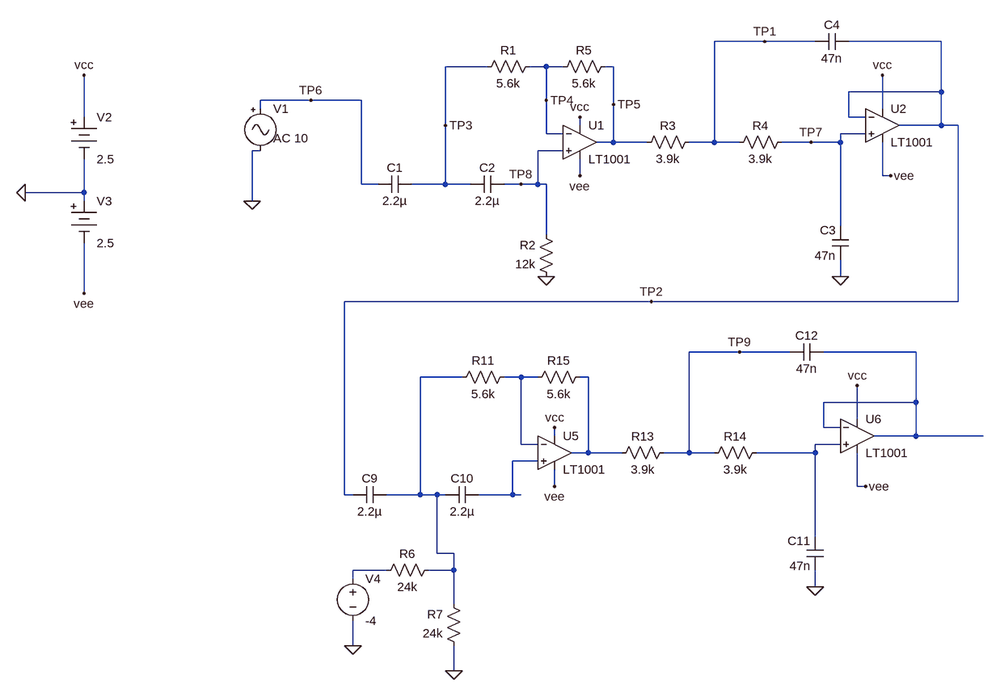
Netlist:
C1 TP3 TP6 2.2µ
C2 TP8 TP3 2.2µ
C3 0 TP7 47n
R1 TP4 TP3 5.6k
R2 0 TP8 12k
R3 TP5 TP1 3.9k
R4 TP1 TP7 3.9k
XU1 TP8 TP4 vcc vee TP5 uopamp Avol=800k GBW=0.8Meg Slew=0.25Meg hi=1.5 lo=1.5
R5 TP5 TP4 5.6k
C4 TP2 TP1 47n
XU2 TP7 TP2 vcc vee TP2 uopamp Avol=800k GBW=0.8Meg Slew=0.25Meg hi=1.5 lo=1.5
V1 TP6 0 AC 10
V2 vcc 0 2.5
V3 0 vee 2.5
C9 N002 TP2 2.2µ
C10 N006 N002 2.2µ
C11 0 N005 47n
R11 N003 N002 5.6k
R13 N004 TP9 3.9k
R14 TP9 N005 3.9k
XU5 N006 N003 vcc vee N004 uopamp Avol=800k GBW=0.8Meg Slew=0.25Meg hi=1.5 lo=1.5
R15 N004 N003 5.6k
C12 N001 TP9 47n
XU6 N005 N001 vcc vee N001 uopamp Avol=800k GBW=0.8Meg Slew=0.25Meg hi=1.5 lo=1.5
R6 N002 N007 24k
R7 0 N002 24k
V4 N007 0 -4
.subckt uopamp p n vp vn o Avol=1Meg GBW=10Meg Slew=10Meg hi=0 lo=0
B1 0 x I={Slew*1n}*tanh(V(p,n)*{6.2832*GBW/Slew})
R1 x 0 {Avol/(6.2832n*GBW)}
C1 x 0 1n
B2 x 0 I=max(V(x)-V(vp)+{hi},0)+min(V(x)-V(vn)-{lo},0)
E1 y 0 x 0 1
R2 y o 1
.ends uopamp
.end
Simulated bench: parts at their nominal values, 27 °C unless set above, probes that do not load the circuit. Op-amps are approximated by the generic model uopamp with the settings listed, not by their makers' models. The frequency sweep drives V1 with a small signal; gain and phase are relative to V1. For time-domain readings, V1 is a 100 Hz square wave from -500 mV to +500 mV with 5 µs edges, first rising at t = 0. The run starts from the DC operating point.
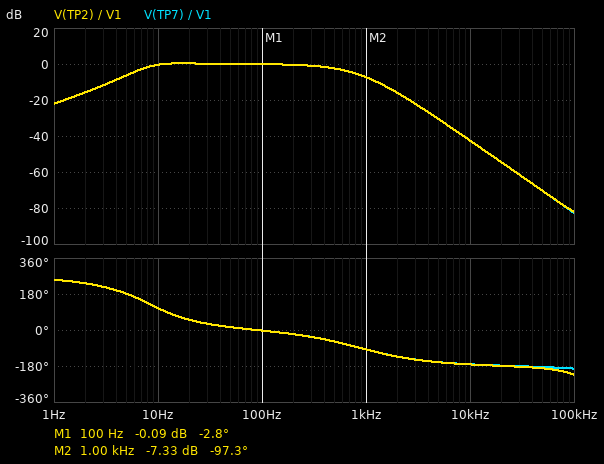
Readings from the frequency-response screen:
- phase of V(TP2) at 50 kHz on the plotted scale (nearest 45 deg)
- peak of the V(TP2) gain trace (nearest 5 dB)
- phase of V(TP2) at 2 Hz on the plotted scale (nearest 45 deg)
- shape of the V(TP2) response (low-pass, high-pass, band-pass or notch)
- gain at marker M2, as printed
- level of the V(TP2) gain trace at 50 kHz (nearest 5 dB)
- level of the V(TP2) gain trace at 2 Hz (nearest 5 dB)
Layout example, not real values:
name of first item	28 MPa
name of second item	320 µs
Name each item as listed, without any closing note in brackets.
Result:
phase of V(TP2) at 50 kHz on the plotted scale	-180 deg
peak of the V(TP2) gain trace	0 dB
phase of V(TP2) at 2 Hz on the plotted scale	225 deg
shape of the V(TP2) response	band-pass
gain at marker M2, as printed	-7.33 dB
level of the V(TP2) gain trace at 50 kHz	-70 dB
level of the V(TP2) gain trace at 2 Hz	-15 dB
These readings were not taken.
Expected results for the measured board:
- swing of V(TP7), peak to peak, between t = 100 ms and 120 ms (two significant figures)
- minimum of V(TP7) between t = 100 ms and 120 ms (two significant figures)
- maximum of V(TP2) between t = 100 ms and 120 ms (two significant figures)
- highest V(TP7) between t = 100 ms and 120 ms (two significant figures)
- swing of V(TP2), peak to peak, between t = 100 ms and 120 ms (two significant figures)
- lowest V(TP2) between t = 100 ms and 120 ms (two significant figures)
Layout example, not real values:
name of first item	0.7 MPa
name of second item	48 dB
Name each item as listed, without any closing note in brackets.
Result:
swing of V(TP7), peak to peak, between t = 100 ms and 120 ms	1.2 V
minimum of V(TP7) between t = 100 ms and 120 ms	-580 mV
maximum of V(TP2) between t = 100 ms and 120 ms	580 mV
highest V(TP7) between t = 100 ms and 120 ms	580 mV
swing of V(TP2), peak to peak, between t = 100 ms and 120 ms	1.2 V
lowest V(TP2) between t = 100 ms and 120 ms	-580 mV
